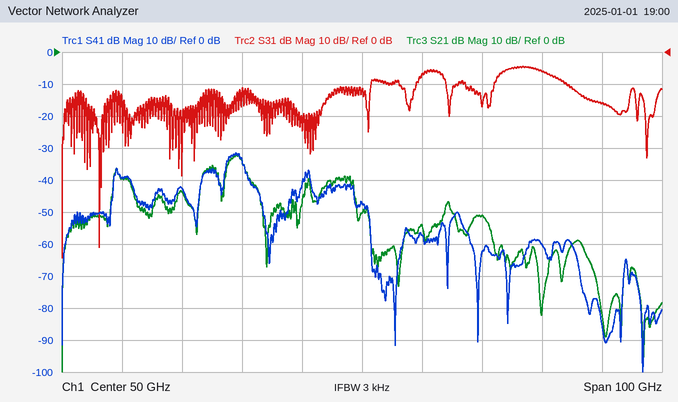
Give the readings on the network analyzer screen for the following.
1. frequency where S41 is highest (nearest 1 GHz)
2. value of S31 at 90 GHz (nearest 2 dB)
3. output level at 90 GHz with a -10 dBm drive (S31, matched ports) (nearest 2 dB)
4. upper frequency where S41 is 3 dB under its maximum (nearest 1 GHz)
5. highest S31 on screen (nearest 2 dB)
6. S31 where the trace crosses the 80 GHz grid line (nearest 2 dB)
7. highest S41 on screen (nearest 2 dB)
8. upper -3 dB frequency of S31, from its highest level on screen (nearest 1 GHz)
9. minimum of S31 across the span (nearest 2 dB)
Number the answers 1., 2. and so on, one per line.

1. 29 GHz
2. -16 dB
3. -26 dBm
4. 30 GHz
5. -4 dB
6. -6 dB
7. -32 dB
8. 82 GHz
9. -64 dB
